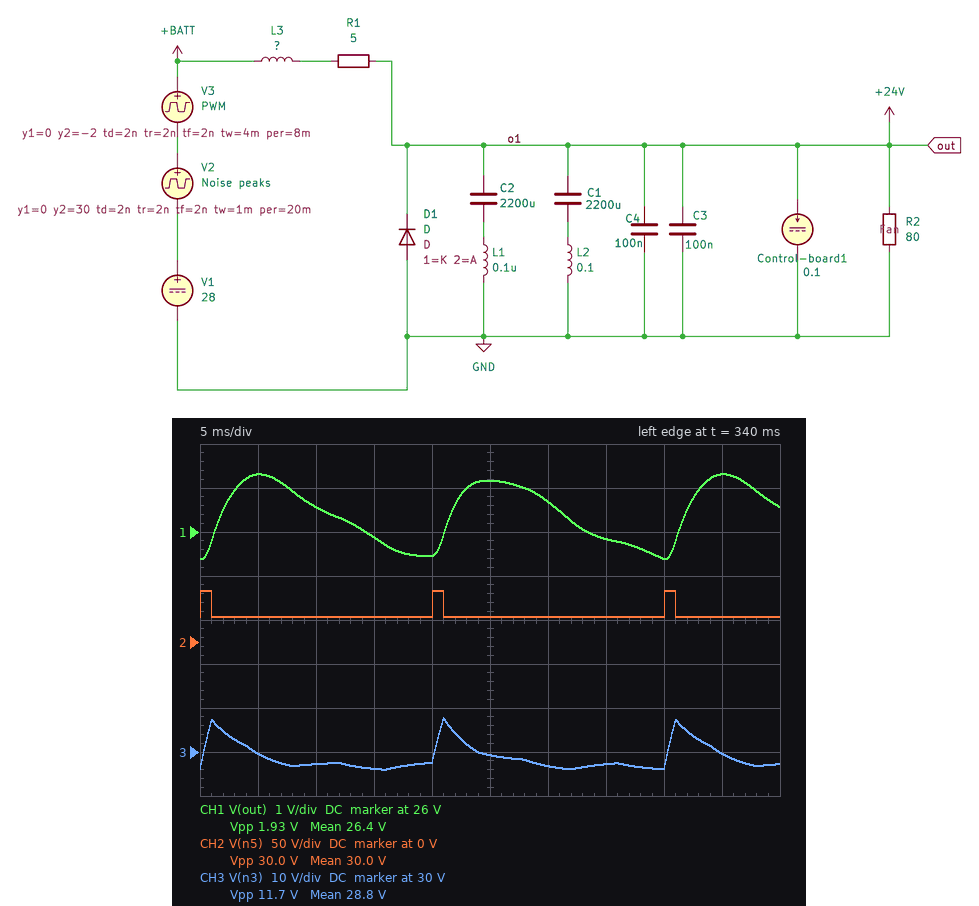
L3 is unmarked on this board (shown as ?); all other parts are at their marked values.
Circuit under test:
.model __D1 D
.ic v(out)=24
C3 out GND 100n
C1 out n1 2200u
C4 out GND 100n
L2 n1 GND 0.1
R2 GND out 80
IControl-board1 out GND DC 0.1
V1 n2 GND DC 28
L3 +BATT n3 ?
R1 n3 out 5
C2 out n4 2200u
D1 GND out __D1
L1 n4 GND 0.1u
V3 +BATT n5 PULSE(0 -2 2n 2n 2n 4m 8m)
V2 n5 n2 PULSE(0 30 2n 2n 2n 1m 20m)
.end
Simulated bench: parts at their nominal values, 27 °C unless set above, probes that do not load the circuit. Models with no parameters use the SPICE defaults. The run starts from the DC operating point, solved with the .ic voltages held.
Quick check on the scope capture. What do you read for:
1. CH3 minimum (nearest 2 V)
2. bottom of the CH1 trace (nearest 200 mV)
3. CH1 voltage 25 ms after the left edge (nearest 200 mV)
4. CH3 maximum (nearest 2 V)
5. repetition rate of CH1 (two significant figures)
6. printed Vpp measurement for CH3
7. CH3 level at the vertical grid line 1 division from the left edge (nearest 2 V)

26 V
25.4 V
27.2 V
38 V
50 Hz
11.7 V
30 V
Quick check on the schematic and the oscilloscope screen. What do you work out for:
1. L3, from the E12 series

12 mH
